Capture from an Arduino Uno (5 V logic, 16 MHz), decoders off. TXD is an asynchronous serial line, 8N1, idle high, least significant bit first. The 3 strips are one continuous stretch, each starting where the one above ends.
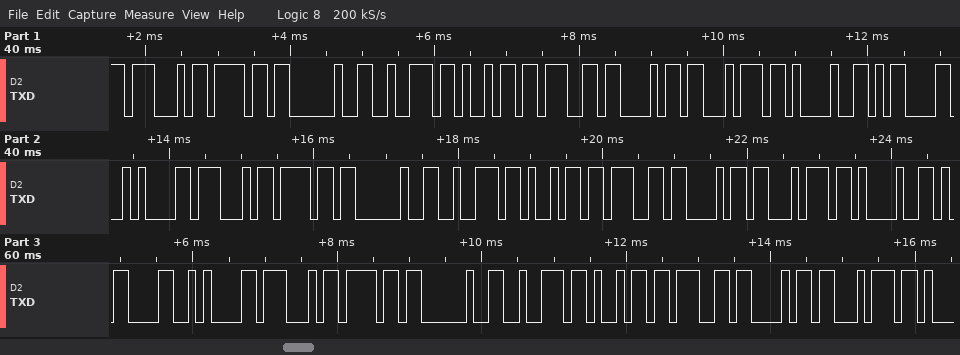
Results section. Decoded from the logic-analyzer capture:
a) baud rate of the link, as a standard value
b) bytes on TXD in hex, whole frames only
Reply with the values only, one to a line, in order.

9600 baud
0x47 0x6F 0x20 0x72 0x69 0x67 0x68 0x74 0x21 0x0D 0x0A 0x47 0x6F 0x20 0x72 0x69 0x67 0x68 0x74 0x21 0x0D 0x0A 0x47 0x6F 0x20 0x72 0x69 0x67 0x68 0x74
